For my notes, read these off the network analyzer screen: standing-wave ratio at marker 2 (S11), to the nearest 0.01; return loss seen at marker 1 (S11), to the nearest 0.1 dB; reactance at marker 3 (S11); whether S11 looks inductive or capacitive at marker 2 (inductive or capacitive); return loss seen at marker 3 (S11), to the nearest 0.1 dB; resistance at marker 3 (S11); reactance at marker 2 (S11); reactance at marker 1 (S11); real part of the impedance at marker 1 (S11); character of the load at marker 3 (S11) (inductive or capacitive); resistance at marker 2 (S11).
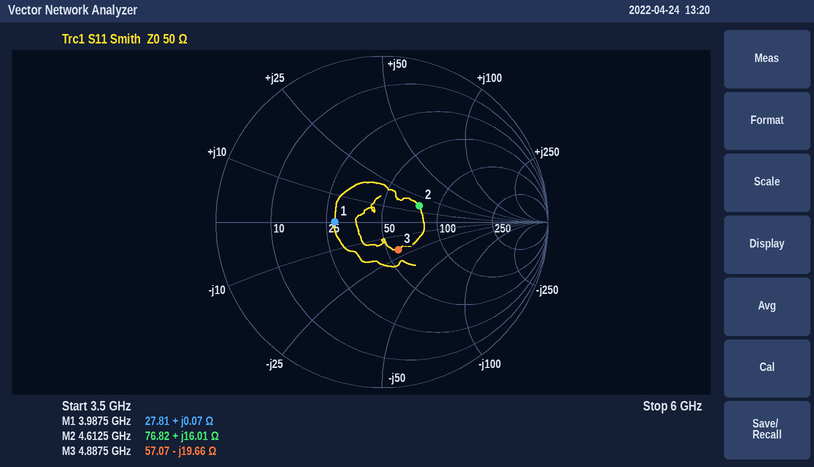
1.65
10.9 dB
-19.66 Ω
inductive
14.3 dB
57.07 Ω
+16.01 Ω
+0.07 Ω
27.81 Ω
capacitive
76.82 Ω
